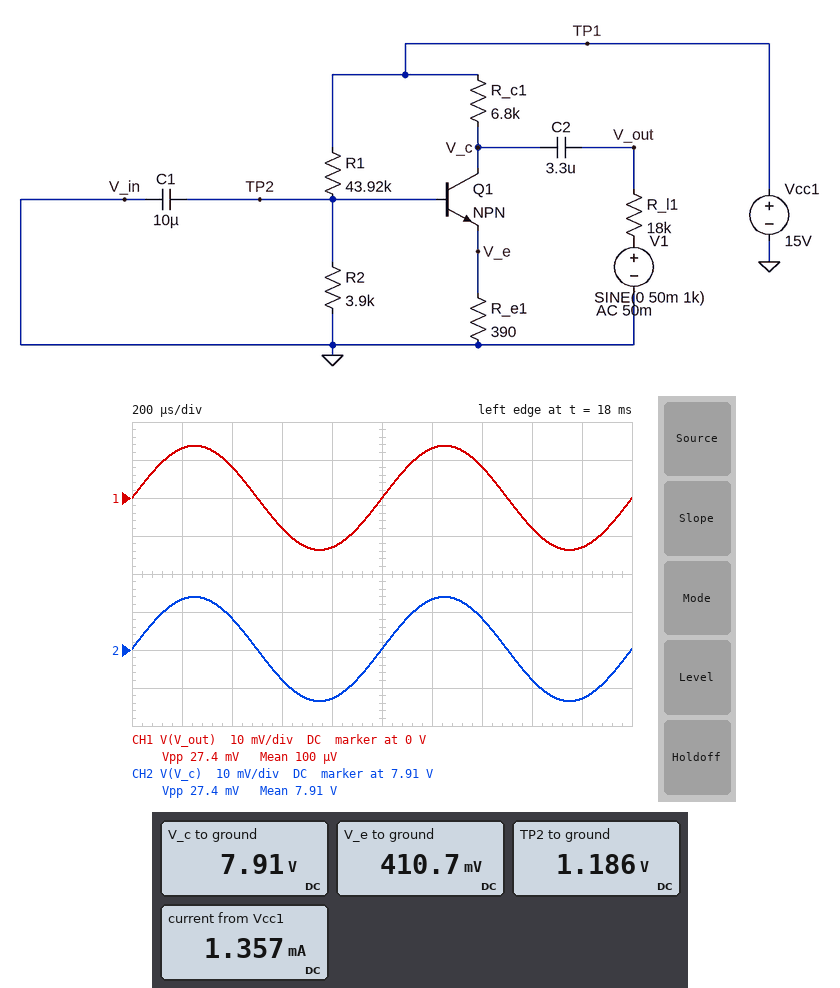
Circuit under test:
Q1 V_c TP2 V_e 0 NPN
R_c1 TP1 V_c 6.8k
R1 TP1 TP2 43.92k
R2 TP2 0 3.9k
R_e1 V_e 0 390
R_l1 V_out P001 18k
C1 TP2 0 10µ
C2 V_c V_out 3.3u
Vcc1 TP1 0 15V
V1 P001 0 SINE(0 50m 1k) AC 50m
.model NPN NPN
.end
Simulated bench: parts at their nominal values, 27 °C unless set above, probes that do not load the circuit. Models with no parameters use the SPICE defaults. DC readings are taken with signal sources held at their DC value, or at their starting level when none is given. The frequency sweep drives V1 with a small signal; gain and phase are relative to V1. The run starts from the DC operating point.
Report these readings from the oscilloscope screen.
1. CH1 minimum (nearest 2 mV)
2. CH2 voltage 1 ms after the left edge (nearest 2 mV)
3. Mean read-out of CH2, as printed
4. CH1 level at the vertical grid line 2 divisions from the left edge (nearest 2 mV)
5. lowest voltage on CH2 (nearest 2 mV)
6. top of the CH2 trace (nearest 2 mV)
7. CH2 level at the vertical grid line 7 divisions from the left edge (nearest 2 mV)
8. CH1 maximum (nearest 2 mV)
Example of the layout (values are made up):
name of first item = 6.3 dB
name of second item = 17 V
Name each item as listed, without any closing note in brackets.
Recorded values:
CH1 minimum = -14 mV
CH2 voltage 1 ms after the left edge = 7.910 V
Mean read-out of CH2, as printed = 7.91 V
CH1 level at the vertical grid line 2 divisions from the left edge = 8 mV
lowest voltage on CH2 = 7.896 V
top of the CH2 trace = 7.924 V
CH2 level at the vertical grid line 7 divisions from the left edge = 7.918 V
CH1 maximum = 14 mV
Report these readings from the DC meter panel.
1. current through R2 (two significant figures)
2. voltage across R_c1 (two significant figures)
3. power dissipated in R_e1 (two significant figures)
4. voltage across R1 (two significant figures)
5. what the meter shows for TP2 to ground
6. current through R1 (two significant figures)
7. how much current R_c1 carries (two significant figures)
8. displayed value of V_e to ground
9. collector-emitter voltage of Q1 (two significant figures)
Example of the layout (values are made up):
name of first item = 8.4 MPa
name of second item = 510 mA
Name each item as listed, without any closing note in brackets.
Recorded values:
current through R2 = 300 µA
voltage across R_c1 = 7.1 V
power dissipated in R_e1 = 430 µW
voltage across R1 = 14 V
what the meter shows for TP2 to ground = 1.186 V
current through R1 = 310 µA
how much current R_c1 carries = 1.0 mA
displayed value of V_e to ground = 410.7 mV
collector-emitter voltage of Q1 = 7.5 V
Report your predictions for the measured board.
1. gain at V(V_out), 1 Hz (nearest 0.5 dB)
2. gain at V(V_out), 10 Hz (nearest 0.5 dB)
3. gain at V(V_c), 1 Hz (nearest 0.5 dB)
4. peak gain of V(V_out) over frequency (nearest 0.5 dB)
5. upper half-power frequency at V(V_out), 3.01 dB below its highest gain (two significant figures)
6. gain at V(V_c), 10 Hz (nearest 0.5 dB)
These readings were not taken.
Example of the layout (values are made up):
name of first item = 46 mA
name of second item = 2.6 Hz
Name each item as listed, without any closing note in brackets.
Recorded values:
gain at V(V_out), 1 Hz = -1.0 dB
gain at V(V_out), 10 Hz = -9.5 dB
gain at V(V_c), 1 Hz = -18.0 dB
peak gain of V(V_out) over frequency = 0 dB
upper half-power frequency at V(V_out), 3.01 dB below its highest gain = 2.1 Hz
gain at V(V_c), 10 Hz = -11.5 dB
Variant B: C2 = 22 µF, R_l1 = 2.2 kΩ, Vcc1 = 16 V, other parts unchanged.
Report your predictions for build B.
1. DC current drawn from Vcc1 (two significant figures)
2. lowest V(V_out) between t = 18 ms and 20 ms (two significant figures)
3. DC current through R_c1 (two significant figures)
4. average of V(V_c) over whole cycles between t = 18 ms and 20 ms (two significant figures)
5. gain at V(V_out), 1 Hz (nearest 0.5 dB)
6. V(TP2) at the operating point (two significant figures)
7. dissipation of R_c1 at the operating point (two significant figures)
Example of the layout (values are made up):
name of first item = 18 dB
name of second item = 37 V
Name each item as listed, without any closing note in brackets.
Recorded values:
DC current drawn from Vcc1 = 1.6 mA
lowest V(V_out) between t = 18 ms and 20 ms = -38 mV
DC current through R_c1 = 1.2 mA
average of V(V_c) over whole cycles between t = 18 ms and 20 ms = 7.7 V
gain at V(V_out), 1 Hz = -1.5 dB
V(TP2) at the operating point = 1.3 V
dissipation of R_c1 at the operating point = 10 mW
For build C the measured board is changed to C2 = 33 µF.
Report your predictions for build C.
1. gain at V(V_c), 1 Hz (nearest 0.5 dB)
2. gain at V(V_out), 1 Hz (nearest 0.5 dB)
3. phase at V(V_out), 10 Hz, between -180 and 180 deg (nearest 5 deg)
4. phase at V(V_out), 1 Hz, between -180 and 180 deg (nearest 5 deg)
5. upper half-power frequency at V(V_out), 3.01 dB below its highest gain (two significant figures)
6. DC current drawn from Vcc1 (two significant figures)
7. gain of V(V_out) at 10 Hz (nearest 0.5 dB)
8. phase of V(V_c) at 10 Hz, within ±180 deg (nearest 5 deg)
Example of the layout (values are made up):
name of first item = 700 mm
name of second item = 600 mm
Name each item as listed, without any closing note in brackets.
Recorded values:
gain at V(V_c), 1 Hz = -11.5 dB
gain at V(V_out), 1 Hz = -9.5 dB
phase at V(V_out), 10 Hz, between -180 and 180 deg = -5 deg
phase at V(V_out), 1 Hz, between -180 and 180 deg = -25 deg
upper half-power frequency at V(V_out), 3.01 dB below its highest gain = 210 mHz
DC current drawn from Vcc1 = 1.4 mA
gain of V(V_out) at 10 Hz = -11.0 dB
phase of V(V_c) at 10 Hz, within ±180 deg = 0 deg
